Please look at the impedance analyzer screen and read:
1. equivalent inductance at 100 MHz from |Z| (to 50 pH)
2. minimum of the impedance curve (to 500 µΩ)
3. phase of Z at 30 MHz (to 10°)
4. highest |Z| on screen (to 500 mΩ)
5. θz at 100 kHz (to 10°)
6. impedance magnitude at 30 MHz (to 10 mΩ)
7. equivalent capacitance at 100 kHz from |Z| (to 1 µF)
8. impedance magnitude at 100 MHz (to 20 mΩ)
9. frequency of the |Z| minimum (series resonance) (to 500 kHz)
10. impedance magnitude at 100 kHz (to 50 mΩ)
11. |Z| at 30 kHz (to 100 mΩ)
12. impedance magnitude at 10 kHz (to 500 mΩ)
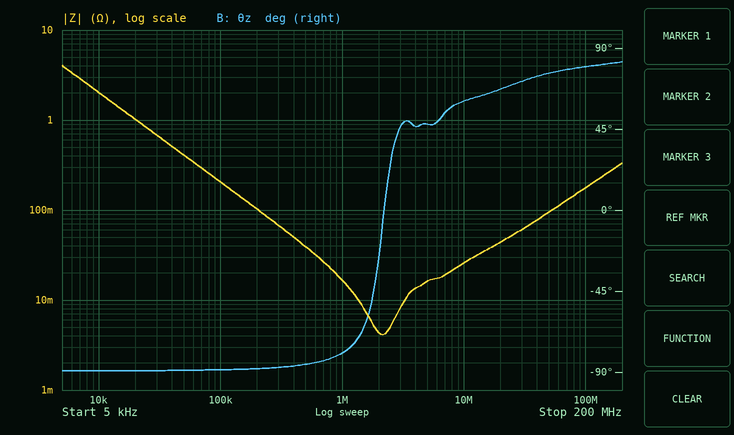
300 pH
4.0 mΩ
70°
4.0 Ω
-90°
60 mΩ
8 µF
180 mΩ
2.0 MHz
200 mΩ
700 mΩ
2.0 Ω
